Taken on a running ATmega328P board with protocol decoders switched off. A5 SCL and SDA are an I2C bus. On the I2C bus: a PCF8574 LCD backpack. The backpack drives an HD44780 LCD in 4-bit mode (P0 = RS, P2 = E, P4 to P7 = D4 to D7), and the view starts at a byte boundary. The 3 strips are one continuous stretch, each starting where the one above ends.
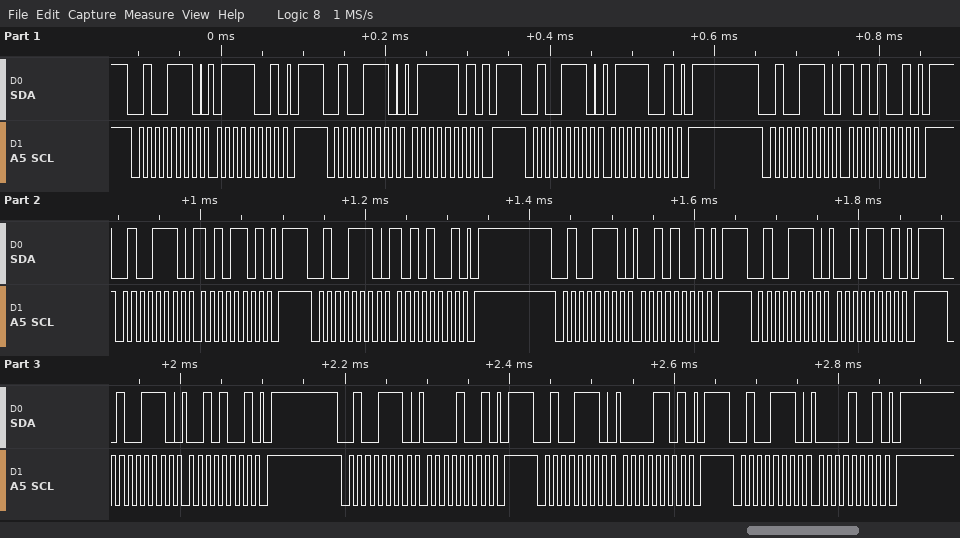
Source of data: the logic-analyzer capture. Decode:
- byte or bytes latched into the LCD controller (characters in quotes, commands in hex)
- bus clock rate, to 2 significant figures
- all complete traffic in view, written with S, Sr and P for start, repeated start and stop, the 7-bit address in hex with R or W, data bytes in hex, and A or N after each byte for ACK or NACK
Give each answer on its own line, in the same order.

'z' ' '
100 kHz
S 27W A 79 A P S 27W A 7D A P S 27W A 79 A P S 27W A A9 A P S 27W A AD A P S 27W A A9 A P S 27W A 29 A P S 27W A 2D A P S 27W A 29 A P S 27W A 09 A P S 27W A 0D A P S 27W A 09 A P
